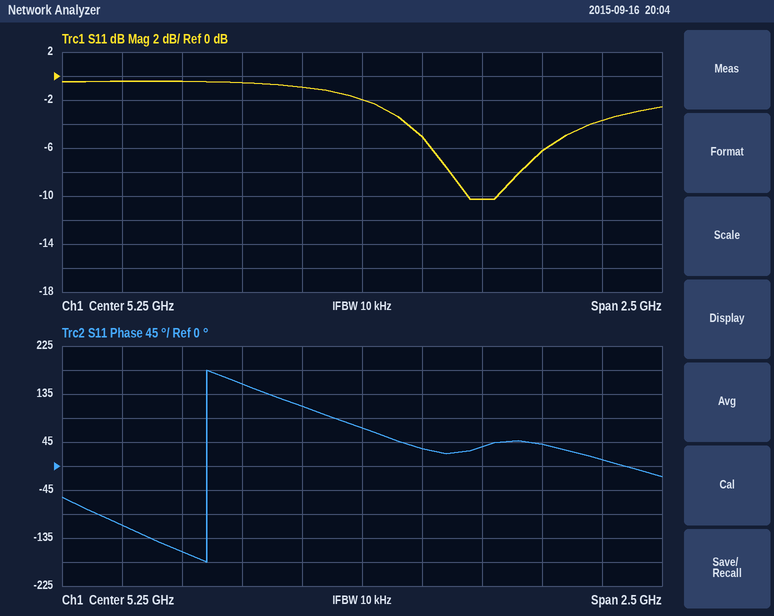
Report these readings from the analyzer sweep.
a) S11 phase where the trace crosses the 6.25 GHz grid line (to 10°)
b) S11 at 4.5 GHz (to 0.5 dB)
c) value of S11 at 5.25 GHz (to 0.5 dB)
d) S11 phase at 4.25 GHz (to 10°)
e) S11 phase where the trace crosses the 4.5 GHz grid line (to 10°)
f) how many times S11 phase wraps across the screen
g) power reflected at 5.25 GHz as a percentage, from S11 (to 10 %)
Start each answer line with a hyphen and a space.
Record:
- 10°
- -0.5 dB
- -2.0 dB
- -110°
- -160°
- 1
- 60 %
